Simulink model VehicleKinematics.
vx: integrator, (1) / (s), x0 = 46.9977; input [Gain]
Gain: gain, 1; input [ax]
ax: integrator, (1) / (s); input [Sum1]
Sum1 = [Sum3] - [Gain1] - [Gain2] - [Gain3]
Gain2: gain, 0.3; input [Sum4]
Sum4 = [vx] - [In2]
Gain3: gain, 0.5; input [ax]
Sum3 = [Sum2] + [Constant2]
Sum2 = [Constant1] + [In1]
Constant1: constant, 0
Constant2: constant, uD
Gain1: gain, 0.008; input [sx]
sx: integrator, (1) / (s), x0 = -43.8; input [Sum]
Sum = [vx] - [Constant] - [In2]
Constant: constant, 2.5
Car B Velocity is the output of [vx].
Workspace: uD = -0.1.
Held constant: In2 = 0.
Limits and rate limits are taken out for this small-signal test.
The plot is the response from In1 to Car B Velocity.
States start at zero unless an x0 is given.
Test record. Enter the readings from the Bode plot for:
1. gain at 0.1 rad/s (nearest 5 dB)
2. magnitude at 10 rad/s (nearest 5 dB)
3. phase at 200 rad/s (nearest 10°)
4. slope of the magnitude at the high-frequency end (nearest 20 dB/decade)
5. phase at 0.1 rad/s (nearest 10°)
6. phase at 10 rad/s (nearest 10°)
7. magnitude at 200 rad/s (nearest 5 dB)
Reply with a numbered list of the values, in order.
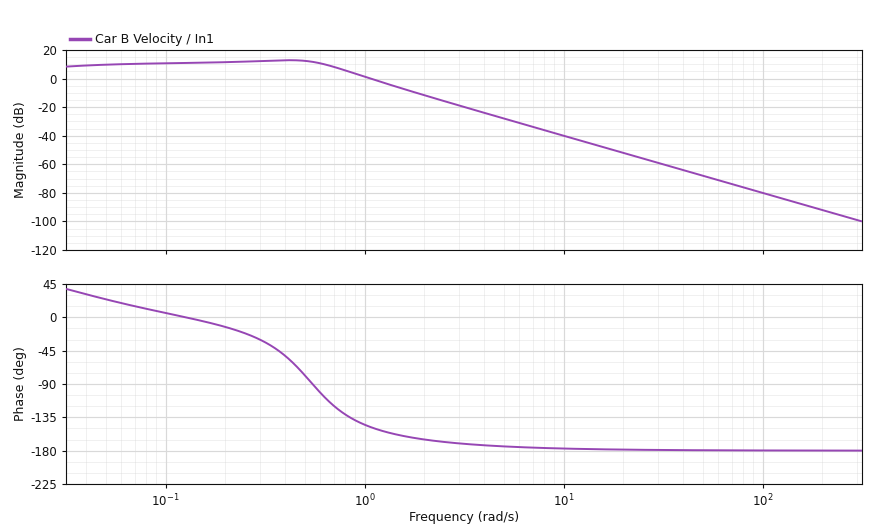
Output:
1. 10 dB
2. -40 dB
3. -180°
4. -40 dB/decade
5. 10°
6. -180°
7. -90 dB
